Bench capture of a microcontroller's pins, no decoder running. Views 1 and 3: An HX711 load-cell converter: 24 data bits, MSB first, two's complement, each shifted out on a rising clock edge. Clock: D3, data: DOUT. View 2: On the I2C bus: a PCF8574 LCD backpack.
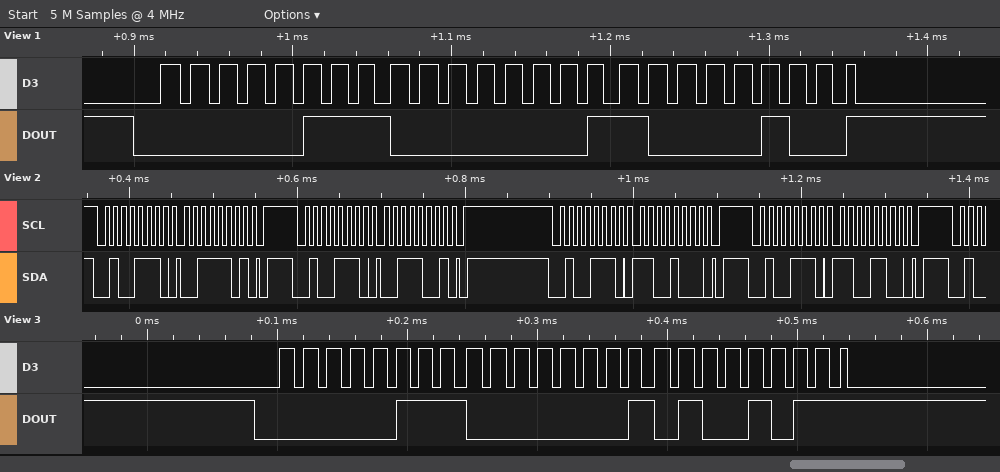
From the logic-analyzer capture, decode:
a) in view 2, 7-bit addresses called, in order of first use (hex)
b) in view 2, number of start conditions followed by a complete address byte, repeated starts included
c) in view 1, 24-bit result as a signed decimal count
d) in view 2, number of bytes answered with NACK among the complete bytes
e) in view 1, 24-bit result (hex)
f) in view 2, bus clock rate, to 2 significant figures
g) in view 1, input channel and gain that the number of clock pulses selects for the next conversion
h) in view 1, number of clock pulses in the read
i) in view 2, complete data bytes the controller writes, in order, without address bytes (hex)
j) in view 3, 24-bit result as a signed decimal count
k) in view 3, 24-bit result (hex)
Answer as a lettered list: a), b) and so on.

a) 0x27
b) 4
c) 459140
d) 0
e) 0x070184
f) 100 kHz
g) channel A, gain 128
h) 25
i) 3D 39 C8 CC
j) 459083
k) 0x07014B
